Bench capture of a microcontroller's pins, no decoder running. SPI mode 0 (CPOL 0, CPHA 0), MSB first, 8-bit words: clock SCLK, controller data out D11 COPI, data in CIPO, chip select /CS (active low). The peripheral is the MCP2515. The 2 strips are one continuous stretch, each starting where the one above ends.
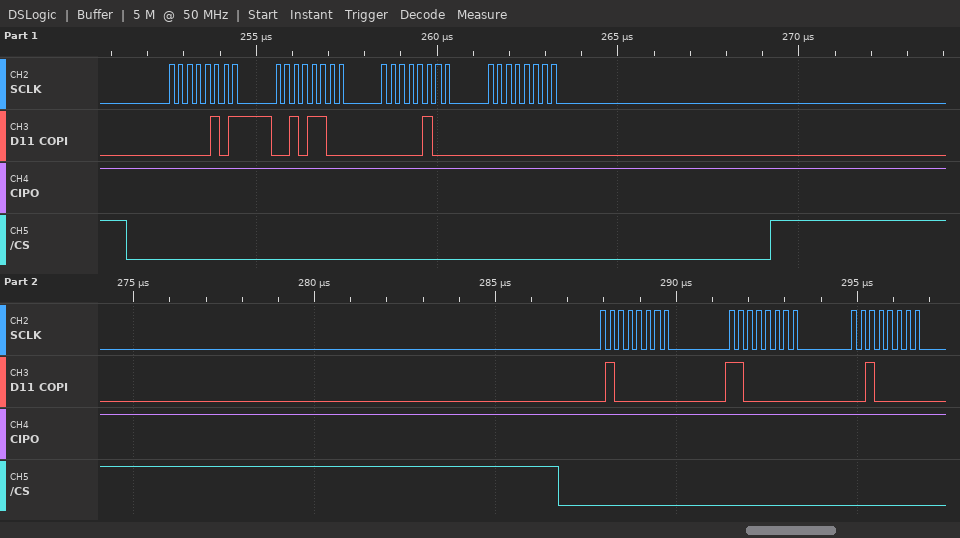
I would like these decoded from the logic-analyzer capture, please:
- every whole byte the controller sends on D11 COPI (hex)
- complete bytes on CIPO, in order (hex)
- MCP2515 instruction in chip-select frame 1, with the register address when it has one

05 2C 04 00 40 C0 20
FF FF FF FF FF FF FF
BIT MODIFY 0x2C
